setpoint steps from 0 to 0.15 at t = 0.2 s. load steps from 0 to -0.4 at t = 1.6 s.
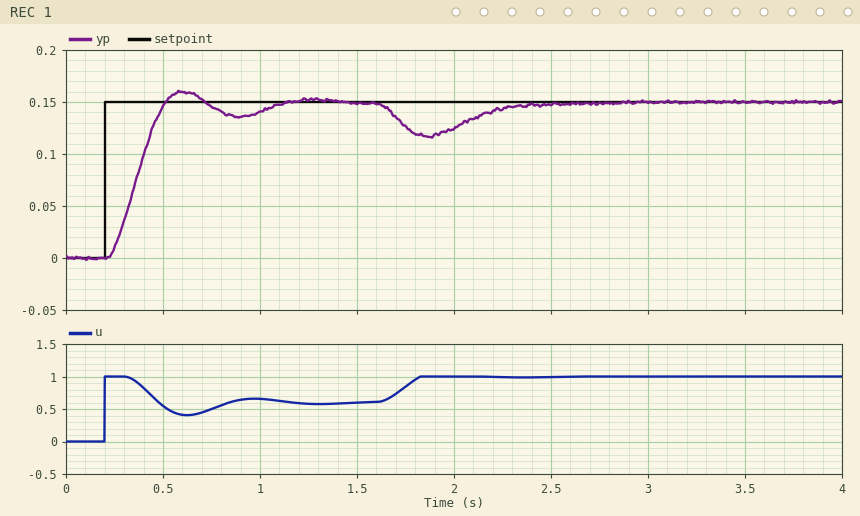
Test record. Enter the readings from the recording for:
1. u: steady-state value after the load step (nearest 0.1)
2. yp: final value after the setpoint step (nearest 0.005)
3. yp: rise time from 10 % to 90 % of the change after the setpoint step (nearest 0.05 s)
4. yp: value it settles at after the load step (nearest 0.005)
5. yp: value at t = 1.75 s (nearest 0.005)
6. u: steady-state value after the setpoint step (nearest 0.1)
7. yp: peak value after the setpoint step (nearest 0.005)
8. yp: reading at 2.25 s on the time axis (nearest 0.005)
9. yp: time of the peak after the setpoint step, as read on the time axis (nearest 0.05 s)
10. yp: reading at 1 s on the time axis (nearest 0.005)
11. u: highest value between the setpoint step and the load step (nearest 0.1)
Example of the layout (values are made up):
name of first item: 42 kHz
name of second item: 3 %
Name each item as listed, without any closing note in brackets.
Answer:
u: steady-state value after the load step: 1.0
yp: final value after the setpoint step: 0.150
yp: rise time from 10 % to 90 % of the change after the setpoint step: 0.20 s
yp: value it settles at after the load step: 0.150
yp: value at t = 1.75 s: 0.125
u: steady-state value after the setpoint step: 0.6
yp: peak value after the setpoint step: 0.160
yp: reading at 2.25 s on the time axis: 0.145
yp: time of the peak after the setpoint step, as read on the time axis: 0.60 s
yp: reading at 1 s on the time axis: 0.140
u: highest value between the setpoint step and the load step: 1.0
